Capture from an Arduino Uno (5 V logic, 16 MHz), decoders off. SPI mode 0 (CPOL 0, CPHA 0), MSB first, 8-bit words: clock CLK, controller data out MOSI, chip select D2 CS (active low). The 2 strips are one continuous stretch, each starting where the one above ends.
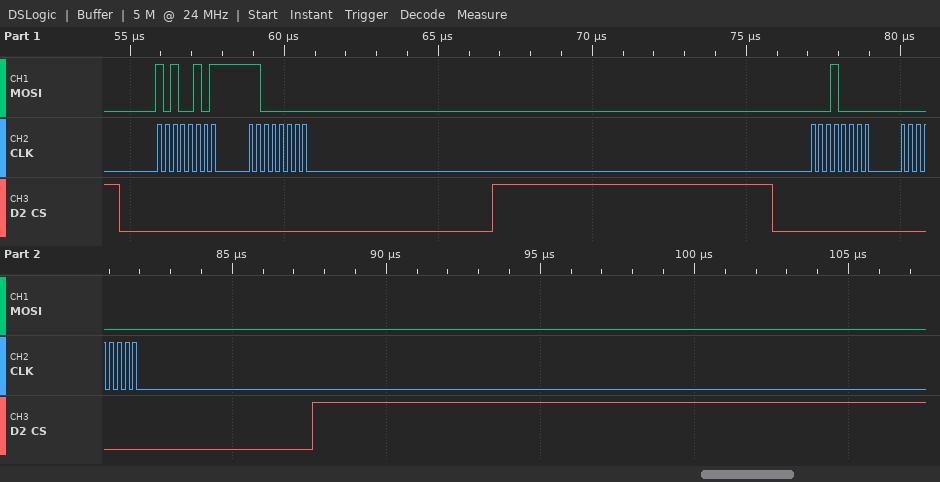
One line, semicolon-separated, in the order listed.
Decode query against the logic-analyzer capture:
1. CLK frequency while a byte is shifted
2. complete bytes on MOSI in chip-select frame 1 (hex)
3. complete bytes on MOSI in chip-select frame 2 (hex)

4 MHz; 0xA5 0xC0; 0x10 0x00
